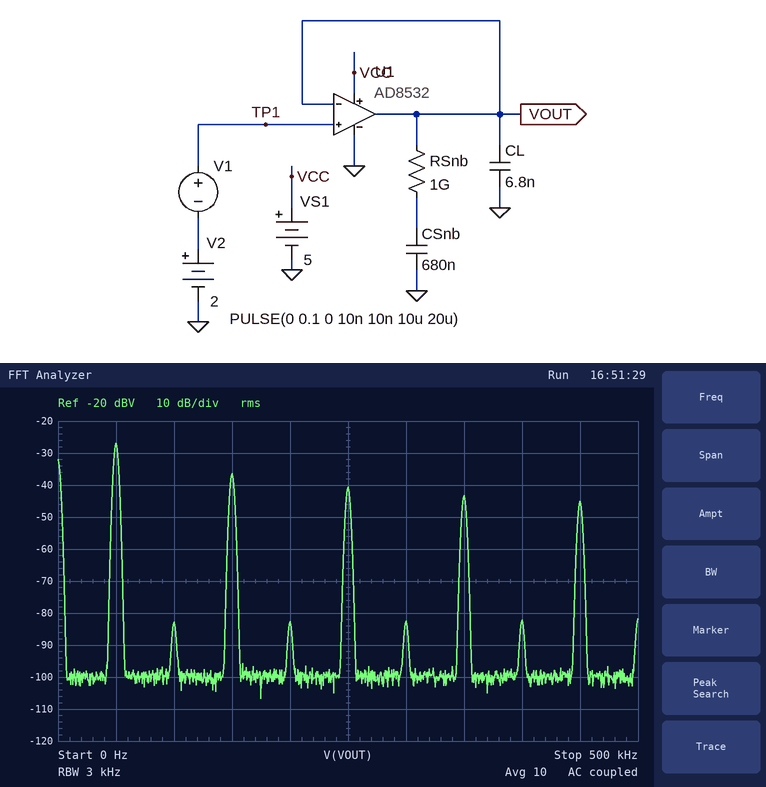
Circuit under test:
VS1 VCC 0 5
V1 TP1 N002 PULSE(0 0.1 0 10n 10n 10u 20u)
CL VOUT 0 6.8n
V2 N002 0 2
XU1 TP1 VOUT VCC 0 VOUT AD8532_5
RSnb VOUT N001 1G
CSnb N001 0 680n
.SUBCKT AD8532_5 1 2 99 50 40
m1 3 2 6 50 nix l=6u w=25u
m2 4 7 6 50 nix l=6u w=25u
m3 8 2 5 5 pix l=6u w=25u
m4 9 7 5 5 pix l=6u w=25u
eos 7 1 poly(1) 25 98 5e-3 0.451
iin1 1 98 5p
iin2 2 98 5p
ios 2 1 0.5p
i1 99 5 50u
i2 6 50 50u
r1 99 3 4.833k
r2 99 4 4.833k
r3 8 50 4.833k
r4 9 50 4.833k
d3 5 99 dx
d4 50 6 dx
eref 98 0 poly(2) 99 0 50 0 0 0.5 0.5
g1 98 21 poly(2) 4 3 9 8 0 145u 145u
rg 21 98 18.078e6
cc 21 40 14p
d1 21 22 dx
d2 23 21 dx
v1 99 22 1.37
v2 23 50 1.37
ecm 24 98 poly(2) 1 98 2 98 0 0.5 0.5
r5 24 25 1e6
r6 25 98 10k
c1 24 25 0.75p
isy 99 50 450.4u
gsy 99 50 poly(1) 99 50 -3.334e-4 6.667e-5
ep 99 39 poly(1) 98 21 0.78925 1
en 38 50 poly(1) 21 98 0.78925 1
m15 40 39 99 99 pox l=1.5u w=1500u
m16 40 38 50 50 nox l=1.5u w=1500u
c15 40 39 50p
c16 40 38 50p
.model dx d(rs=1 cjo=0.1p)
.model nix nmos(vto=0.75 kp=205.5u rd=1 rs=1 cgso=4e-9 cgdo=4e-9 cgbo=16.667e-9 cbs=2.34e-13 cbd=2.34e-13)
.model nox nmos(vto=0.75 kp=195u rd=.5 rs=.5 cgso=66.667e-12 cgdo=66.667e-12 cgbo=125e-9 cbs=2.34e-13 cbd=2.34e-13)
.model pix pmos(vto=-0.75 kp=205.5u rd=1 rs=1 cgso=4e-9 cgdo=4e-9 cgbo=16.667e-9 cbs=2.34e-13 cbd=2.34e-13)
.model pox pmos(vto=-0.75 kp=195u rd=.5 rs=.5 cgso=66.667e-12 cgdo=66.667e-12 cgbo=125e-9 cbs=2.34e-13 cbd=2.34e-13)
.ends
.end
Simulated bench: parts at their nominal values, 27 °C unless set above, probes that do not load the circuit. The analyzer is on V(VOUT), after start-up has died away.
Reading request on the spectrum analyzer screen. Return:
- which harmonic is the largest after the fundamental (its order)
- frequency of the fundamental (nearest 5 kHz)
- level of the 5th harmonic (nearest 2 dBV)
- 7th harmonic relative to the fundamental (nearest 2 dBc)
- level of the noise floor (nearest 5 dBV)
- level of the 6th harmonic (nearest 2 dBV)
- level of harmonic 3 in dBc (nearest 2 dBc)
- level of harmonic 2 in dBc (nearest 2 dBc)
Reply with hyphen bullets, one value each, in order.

- 3
- 50 kHz
- -40 dBV
- -16 dBc
- -100 dBV
- -82 dBV
- -10 dBc
- -56 dBc
